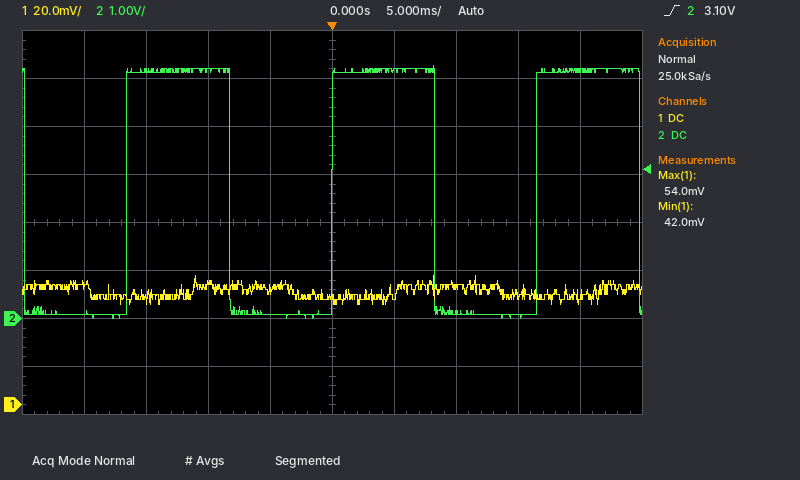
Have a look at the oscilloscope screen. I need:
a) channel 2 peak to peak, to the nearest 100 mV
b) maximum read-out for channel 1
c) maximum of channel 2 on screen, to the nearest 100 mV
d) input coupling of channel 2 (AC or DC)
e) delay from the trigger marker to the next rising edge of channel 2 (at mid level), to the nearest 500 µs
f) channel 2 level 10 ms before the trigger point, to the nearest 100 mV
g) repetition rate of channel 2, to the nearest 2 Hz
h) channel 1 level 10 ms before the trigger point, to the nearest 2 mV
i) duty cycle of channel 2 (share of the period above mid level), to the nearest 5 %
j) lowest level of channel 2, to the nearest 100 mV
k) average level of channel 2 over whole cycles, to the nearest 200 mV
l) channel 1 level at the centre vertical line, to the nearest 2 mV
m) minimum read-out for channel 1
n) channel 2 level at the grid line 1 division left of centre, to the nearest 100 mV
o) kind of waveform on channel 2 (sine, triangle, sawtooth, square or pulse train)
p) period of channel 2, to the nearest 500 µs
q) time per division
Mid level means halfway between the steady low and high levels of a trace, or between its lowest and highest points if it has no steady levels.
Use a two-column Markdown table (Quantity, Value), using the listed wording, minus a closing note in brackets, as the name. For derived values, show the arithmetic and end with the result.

| Quantity | Value |
|---|---|
| channel 2 peak to peak, to the nearest 100 mV | 5.3 V − (0.0 V) = 5.3 V |
| maximum read-out for channel 1 | 54.0 mV |
| maximum of channel 2 on screen, to the nearest 100 mV | 5.3 V |
| input coupling of channel 2 | DC |
| delay from the trigger marker to the next rising edge of channel 2 (at mid level), to the nearest 500 µs | 16.5 ms |
| channel 2 level 10 ms before the trigger point, to the nearest 100 mV | 5.2 V |
| repetition rate of channel 2, to the nearest 2 Hz | 1 / 16.5 ms ≈ 60.6 Hz, so 60 Hz to the nearest 2 Hz |
| channel 1 level 10 ms before the trigger point, to the nearest 2 mV | 50 mV |
| duty cycle of channel 2 (share of the period above mid level), to the nearest 5 % | 50 % |
| lowest level of channel 2, to the nearest 100 mV | 0.0 V |
| average level of channel 2 over whole cycles, to the nearest 200 mV | 0.0 V + 0.5 × (5.3 V − (0.0 V)) ≈ 2.6 V |
| channel 1 level at the centre vertical line, to the nearest 2 mV | 44 mV |
| minimum read-out for channel 1 | 42.0 mV |
| channel 2 level at the grid line 1 division left of centre, to the nearest 100 mV | 100 mV |
| kind of waveform on channel 2 | square |
| period of channel 2, to the nearest 500 µs | 16.5 ms |
| time per division | 5 ms |
